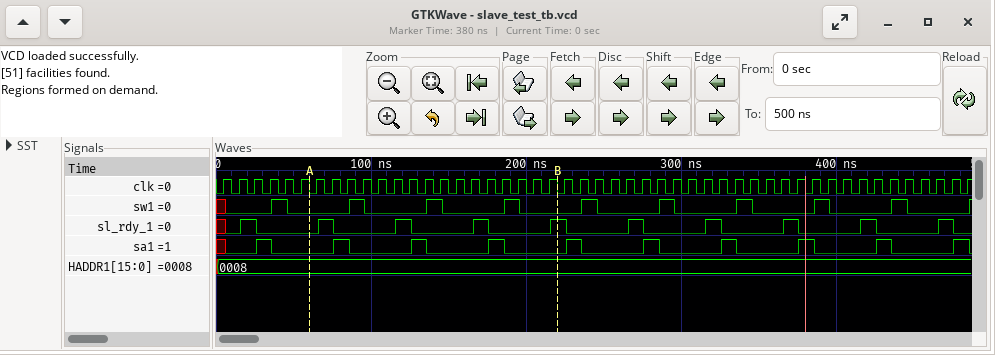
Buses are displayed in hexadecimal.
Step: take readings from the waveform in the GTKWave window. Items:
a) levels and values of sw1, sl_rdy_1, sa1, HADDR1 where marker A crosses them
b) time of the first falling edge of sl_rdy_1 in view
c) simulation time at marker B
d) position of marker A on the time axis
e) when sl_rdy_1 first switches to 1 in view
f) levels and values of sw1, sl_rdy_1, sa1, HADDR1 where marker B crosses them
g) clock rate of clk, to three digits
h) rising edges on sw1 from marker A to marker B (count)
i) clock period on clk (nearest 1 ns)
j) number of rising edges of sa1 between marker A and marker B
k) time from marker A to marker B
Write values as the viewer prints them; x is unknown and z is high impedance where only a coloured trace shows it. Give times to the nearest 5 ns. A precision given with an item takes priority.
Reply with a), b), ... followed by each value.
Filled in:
a) sw1=0, sl_rdy_1=0, sa1=0, HADDR1=0008
b) 25 ns
c) 220 ns
d) 60 ns
e) 15 ns
f) sw1=0, sl_rdy_1=1, sa1=0, HADDR1=0008
g) 100 MHz
h) 3
i) 10 ns
j) 3
k) 160 ns
